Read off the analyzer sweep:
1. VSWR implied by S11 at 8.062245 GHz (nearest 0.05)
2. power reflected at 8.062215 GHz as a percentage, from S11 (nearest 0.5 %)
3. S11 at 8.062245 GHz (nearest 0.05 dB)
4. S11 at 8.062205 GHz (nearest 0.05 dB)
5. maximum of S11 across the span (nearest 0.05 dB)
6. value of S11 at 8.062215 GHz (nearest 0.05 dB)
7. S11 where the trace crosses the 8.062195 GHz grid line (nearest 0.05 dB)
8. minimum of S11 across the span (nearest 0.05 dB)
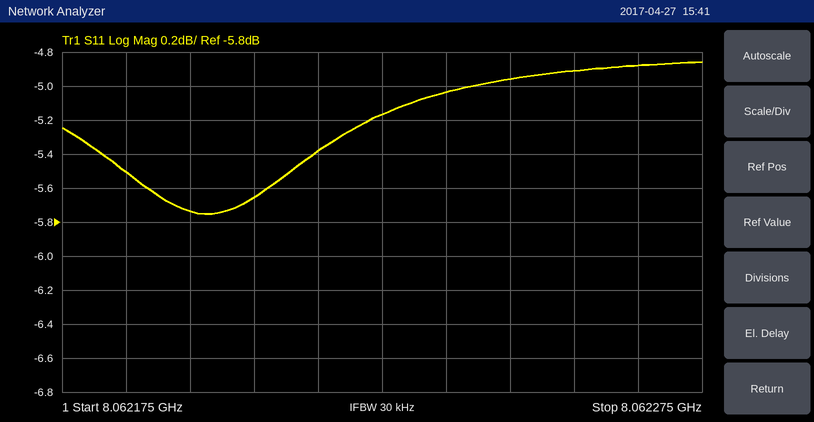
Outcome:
3.60
29.0 %
-4.95 dB
-5.65 dB
-4.85 dB
-5.40 dB
-5.75 dB
-5.75 dB
